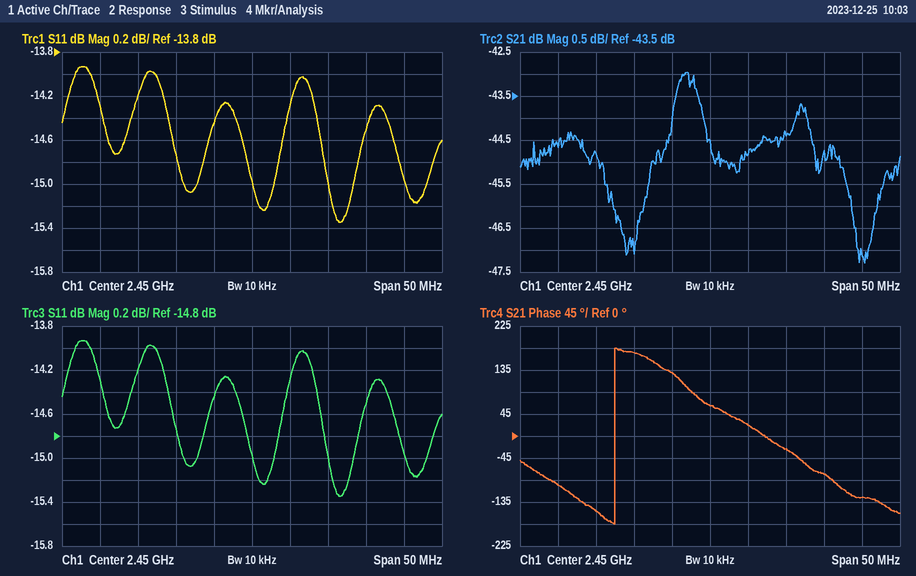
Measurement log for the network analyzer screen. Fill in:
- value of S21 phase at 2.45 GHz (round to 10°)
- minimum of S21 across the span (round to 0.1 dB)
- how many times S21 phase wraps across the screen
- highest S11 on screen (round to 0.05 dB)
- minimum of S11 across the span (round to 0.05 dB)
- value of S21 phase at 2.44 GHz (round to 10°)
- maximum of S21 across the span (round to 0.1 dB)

60°
-47.3 dB
1
-13.95 dB
-15.35 dB
170°
-43.0 dB
